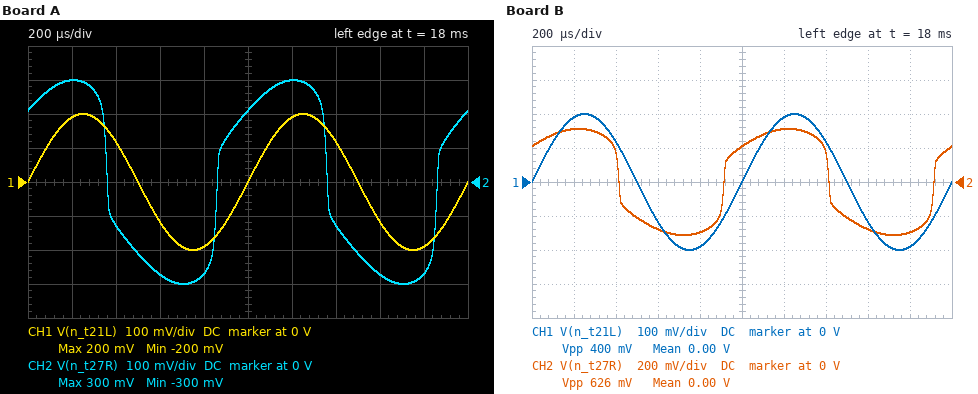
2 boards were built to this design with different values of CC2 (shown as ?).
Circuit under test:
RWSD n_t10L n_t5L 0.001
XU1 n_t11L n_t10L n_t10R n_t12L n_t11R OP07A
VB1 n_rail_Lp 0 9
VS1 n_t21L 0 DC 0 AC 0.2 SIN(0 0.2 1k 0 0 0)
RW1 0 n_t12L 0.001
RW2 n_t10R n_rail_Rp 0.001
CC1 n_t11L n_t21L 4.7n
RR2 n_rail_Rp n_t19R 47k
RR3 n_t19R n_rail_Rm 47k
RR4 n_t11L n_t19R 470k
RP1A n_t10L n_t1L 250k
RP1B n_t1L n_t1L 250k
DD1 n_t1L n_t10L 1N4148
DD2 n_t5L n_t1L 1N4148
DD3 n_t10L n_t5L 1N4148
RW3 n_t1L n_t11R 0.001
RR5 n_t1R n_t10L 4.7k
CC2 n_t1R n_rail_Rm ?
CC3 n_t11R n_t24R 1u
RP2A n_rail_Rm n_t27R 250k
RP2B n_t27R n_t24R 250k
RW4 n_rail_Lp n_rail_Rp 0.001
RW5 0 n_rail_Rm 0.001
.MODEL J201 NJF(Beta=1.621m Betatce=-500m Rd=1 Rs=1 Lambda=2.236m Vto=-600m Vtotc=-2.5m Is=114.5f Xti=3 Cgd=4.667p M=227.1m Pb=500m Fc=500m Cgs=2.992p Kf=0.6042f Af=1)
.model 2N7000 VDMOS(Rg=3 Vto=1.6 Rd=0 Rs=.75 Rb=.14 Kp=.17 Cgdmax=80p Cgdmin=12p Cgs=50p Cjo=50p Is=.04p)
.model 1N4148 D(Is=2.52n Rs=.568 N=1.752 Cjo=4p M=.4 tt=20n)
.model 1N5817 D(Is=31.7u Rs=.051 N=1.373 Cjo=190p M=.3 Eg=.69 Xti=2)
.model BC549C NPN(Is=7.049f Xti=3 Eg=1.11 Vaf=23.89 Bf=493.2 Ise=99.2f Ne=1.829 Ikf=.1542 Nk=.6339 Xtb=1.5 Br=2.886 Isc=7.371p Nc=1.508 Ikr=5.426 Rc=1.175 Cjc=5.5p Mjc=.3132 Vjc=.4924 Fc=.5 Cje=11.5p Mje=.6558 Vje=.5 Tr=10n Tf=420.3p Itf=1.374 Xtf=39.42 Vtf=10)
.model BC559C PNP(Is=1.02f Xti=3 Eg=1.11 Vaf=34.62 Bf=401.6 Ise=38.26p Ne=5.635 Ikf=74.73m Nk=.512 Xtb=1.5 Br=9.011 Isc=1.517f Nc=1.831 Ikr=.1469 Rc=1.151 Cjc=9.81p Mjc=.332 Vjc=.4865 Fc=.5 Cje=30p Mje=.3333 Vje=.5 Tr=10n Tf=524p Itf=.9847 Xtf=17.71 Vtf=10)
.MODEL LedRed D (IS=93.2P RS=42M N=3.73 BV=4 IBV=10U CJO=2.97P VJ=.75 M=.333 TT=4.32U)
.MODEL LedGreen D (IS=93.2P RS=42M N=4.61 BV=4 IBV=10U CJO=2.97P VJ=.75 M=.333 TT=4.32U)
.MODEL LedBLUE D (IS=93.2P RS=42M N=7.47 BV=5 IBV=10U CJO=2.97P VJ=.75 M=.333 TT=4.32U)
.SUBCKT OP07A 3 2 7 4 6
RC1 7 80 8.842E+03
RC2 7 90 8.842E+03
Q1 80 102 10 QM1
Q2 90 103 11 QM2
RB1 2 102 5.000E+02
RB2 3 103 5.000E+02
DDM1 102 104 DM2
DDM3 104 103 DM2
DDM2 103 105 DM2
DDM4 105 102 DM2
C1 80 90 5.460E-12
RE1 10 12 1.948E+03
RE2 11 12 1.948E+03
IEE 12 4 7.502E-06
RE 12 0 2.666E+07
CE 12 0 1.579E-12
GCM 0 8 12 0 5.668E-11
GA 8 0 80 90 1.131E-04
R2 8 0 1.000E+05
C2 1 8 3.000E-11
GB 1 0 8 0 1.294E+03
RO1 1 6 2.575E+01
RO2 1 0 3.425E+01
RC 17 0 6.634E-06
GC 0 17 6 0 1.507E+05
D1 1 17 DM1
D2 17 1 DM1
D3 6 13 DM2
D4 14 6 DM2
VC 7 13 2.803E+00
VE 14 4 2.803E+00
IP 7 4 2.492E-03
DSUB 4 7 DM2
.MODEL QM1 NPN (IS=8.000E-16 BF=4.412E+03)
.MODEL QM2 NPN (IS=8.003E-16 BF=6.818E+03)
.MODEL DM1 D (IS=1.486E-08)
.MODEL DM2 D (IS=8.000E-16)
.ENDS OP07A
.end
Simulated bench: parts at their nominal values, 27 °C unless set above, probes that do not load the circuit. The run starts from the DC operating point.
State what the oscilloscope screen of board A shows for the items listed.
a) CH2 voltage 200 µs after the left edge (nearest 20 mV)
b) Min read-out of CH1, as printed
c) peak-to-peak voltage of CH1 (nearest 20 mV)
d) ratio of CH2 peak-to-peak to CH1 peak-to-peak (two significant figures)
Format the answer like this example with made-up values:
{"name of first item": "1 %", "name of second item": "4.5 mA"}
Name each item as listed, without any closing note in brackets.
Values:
{"CH2 voltage 200 µs after the left edge": "300 mV", "Min read-out of CH1, as printed": "-200 mV", "peak-to-peak voltage of CH1": "400 mV", "ratio of CH2 peak-to-peak to CH1 peak-to-peak": "1.5"}
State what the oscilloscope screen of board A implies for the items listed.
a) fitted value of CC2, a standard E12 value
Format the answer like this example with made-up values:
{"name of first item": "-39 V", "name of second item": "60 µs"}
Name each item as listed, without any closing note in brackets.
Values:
{"fitted value of CC2, a standard E12 value": "27 nF"}
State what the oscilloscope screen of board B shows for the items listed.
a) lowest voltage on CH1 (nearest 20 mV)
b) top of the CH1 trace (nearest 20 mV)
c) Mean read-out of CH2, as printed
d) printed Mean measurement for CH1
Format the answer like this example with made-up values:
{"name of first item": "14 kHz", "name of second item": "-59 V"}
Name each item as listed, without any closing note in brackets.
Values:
{"lowest voltage on CH1": "-200 mV", "top of the CH1 trace": "200 mV", "Mean read-out of CH2, as printed": "0.00 V", "printed Mean measurement for CH1": "0.00 V"}
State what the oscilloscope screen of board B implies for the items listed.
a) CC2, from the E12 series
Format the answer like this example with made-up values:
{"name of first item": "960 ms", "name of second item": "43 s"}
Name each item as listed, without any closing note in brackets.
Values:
{"CC2, from the E12 series": "56 nF"}
